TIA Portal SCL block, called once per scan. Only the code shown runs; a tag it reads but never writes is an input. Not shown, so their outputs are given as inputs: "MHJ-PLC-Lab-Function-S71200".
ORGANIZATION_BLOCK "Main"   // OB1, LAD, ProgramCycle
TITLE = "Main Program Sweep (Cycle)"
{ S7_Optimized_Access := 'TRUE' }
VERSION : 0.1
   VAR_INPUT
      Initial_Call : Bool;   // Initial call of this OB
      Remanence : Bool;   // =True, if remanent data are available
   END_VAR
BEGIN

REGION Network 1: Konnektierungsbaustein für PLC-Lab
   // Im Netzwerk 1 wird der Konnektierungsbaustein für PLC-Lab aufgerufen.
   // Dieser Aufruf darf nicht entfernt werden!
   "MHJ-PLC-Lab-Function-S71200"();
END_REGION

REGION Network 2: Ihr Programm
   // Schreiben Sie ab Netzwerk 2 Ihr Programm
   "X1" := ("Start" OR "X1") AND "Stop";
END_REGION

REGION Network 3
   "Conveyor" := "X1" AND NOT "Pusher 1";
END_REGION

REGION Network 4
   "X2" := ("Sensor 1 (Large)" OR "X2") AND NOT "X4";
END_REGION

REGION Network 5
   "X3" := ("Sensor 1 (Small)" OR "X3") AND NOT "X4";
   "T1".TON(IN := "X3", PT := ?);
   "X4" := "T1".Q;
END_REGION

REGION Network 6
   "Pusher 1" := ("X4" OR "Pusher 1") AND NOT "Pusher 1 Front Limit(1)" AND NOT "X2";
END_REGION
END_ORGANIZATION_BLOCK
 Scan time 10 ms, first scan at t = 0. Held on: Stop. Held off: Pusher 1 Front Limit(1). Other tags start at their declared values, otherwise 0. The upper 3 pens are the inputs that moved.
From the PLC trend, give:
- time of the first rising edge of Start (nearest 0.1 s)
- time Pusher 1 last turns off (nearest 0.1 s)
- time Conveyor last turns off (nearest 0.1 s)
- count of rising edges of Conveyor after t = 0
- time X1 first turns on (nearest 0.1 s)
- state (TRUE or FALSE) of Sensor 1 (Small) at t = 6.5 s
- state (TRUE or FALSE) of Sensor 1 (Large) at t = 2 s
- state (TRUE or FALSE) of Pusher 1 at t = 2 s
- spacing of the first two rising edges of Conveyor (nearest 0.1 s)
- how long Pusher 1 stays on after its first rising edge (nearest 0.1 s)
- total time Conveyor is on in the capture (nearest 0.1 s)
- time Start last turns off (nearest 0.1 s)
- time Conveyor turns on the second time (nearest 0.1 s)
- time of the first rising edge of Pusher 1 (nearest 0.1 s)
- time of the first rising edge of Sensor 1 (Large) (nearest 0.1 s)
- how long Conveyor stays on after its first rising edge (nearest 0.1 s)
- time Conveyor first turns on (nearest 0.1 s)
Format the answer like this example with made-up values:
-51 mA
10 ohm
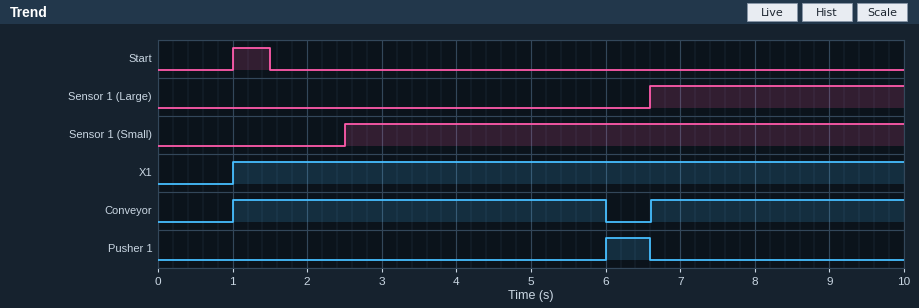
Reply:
1.0 s
6.6 s
6.0 s
2
1.0 s
TRUE
FALSE
FALSE
5.6 s
0.6 s
8.4 s
1.5 s
6.6 s
6.0 s
6.6 s
5.0 s
1.0 s
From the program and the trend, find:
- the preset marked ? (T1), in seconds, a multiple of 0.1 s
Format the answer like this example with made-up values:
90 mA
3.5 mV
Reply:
3.5 s
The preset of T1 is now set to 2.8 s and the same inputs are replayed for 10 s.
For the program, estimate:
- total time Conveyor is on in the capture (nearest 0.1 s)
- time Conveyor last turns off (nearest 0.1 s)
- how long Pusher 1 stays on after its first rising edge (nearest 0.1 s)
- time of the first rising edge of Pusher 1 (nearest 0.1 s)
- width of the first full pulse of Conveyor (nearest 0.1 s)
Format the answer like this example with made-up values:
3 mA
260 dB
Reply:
7.7 s
5.3 s
1.3 s
5.3 s
4.3 s
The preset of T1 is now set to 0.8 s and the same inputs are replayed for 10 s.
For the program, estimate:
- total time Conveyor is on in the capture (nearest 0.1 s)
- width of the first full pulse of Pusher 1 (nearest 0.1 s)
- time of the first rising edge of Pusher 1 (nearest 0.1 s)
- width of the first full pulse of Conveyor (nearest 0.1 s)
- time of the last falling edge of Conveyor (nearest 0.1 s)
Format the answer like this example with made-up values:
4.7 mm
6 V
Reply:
5.7 s
3.3 s
3.3 s
2.3 s
3.3 s
